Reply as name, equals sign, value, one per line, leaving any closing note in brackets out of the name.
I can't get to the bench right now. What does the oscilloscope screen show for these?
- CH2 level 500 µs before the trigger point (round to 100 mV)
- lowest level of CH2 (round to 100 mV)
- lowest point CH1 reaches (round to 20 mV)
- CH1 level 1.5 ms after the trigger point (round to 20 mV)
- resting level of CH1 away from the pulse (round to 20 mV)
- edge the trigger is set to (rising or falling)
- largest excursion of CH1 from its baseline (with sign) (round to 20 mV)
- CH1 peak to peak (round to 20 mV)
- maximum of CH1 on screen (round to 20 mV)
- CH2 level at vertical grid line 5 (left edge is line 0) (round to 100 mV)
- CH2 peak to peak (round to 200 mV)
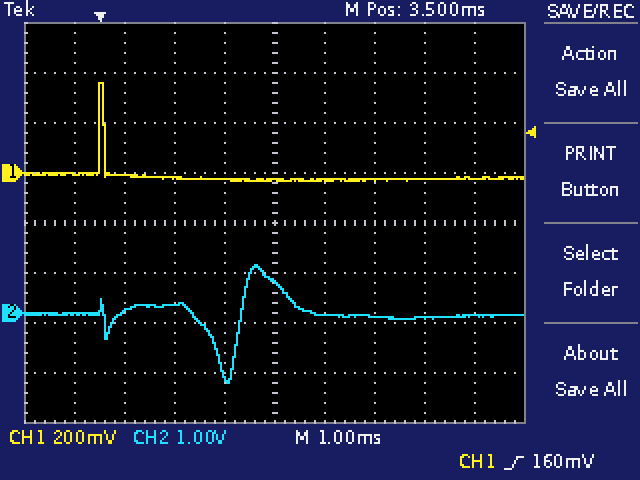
CH2 level 500 µs before the trigger point = 0.0 V
lowest level of CH2 = -1.4 V
lowest point CH1 reaches = -40 mV
CH1 level 1.5 ms after the trigger point = -20 mV
resting level of CH1 away from the pulse = -20 mV
edge the trigger is set to = rising
largest excursion of CH1 from its baseline (with sign) = +380 mV
CH1 peak to peak = 400 mV
maximum of CH1 on screen = 360 mV
CH2 level at vertical grid line 5 (left edge is line 0) = 600 mV
CH2 peak to peak = 2.4 V
